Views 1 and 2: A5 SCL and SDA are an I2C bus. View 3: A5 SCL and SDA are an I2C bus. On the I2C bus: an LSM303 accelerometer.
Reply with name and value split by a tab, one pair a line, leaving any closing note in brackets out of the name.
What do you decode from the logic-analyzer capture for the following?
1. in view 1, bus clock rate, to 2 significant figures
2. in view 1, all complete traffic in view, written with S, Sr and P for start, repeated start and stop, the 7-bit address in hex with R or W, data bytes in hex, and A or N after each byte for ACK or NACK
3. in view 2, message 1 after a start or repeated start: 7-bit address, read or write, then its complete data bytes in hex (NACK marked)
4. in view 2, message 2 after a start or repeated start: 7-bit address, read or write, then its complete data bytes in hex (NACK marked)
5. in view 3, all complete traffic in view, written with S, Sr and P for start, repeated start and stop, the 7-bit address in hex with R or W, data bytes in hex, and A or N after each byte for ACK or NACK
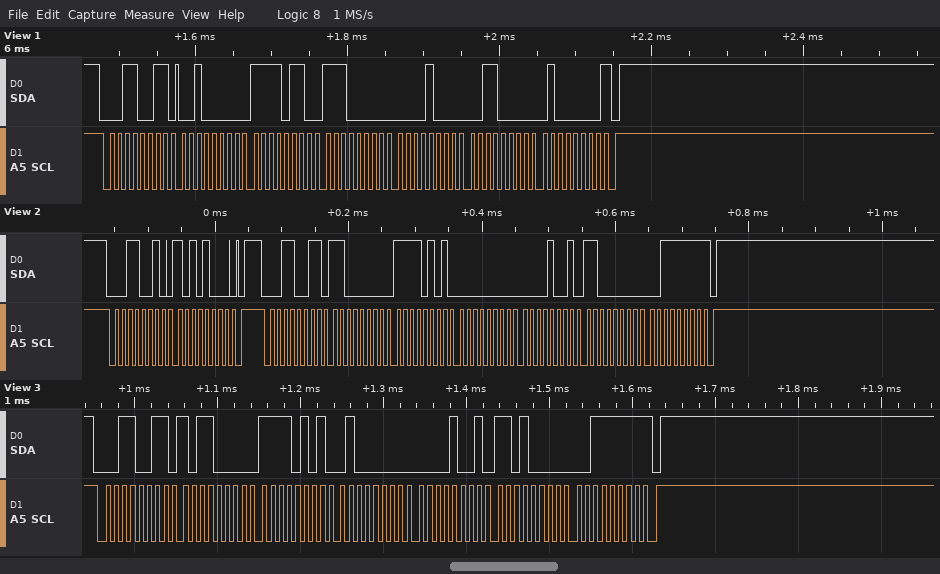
in view 1, bus clock rate, to 2 significant figures	100 kHz
in view 1, all complete traffic in view, written with S, Sr and P for start, repeated start and stop, the 7-bit address in hex with R or W, data bytes in hex, and A or N after each byte for ACK or NACK	S 19R A 20 A F6 A E0 A 08 A 30 A 40 N P
in view 2, message 1 after a start or repeated start: 7-bit address, read or write, then its complete data bytes in hex	0x19 write: A8
in view 2, message 2 after a start or repeated start: 7-bit address, read or write, then its complete data bytes in hex	0x19 read: C0 F5 00 09 C0 3F NACK
in view 3, all complete traffic in view, written with S, Sr and P for start, repeated start and stop, the 7-bit address in hex with R or W, data bytes in hex, and A or N after each byte for ACK or NACK	S 19R A B0 A F5 A 40 A 09 A D0 A 3F N P
